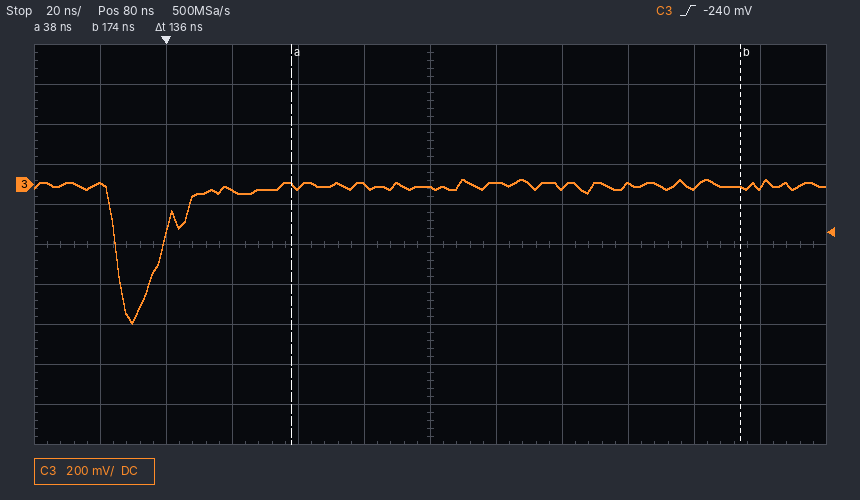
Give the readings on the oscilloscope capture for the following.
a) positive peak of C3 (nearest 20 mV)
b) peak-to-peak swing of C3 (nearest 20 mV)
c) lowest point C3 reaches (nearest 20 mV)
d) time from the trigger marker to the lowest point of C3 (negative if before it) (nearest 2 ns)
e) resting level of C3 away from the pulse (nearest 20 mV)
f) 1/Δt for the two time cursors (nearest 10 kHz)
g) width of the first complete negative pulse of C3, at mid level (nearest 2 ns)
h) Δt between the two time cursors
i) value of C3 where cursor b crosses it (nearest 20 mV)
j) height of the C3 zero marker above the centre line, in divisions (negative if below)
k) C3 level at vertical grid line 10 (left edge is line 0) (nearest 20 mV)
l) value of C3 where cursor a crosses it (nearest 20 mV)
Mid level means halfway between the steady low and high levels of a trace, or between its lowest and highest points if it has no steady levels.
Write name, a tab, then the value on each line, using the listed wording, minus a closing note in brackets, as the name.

positive peak of C3	20 mV
peak-to-peak swing of C3	720 mV
lowest point C3 reaches	-700 mV
time from the trigger marker to the lowest point of C3 (negative if before it)	-10 ns
resting level of C3 away from the pulse	0 mV
1/Δt for the two time cursors	7.35 MHz
width of the first complete negative pulse of C3, at mid level	14 ns
Δt between the two time cursors	136 ns
value of C3 where cursor b crosses it	-20 mV
height of the C3 zero marker above the centre line, in divisions	+1.5 div
C3 level at vertical grid line 10 (left edge is line 0)	-20 mV
value of C3 where cursor a crosses it	0 mV
